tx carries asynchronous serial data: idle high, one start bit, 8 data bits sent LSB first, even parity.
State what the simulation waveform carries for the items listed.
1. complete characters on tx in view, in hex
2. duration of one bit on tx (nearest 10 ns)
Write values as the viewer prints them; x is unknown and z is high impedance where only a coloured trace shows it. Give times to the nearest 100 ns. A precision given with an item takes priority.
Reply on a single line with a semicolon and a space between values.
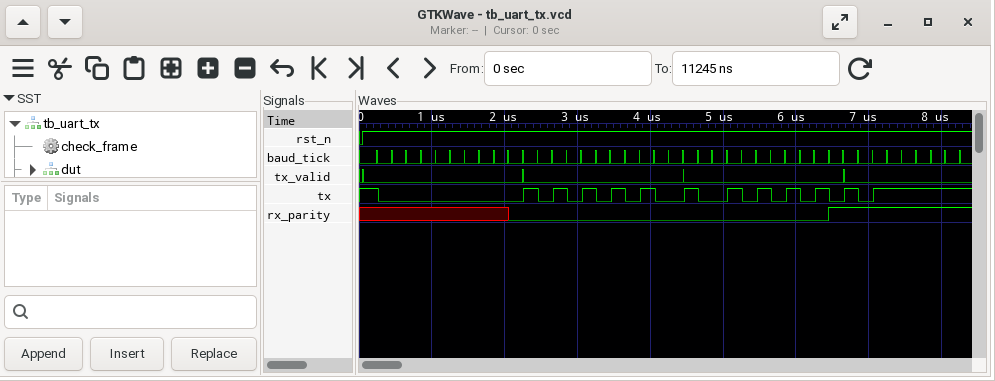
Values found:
00, 55, AA; 200 ns
